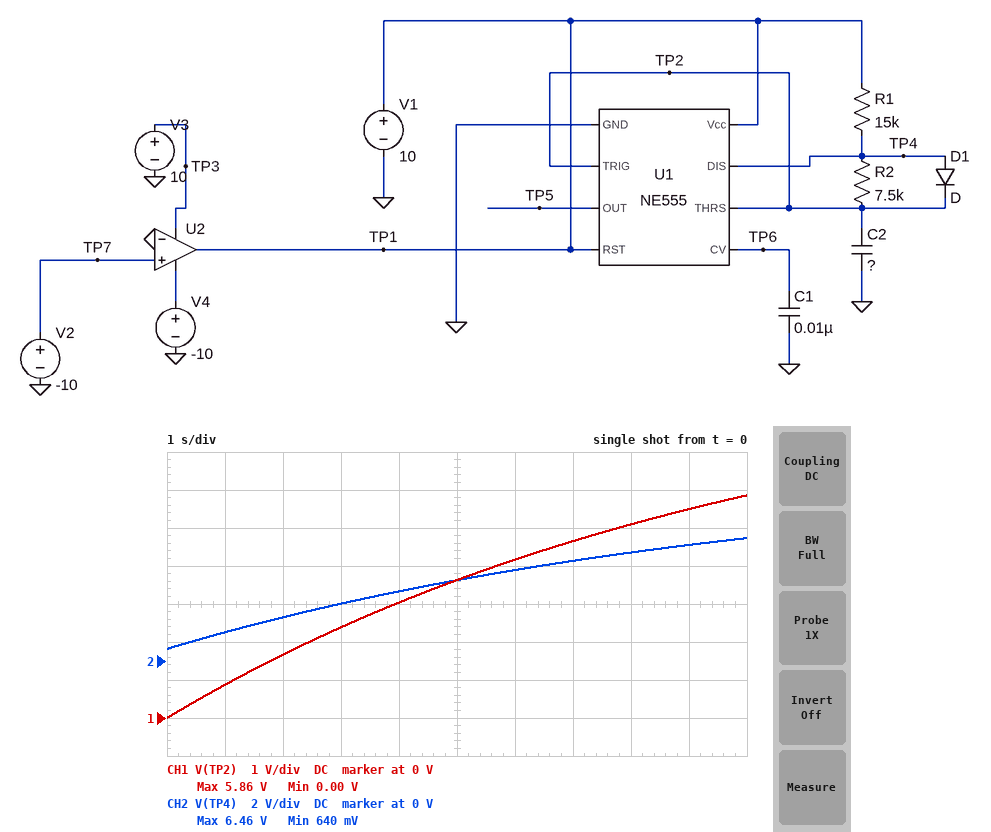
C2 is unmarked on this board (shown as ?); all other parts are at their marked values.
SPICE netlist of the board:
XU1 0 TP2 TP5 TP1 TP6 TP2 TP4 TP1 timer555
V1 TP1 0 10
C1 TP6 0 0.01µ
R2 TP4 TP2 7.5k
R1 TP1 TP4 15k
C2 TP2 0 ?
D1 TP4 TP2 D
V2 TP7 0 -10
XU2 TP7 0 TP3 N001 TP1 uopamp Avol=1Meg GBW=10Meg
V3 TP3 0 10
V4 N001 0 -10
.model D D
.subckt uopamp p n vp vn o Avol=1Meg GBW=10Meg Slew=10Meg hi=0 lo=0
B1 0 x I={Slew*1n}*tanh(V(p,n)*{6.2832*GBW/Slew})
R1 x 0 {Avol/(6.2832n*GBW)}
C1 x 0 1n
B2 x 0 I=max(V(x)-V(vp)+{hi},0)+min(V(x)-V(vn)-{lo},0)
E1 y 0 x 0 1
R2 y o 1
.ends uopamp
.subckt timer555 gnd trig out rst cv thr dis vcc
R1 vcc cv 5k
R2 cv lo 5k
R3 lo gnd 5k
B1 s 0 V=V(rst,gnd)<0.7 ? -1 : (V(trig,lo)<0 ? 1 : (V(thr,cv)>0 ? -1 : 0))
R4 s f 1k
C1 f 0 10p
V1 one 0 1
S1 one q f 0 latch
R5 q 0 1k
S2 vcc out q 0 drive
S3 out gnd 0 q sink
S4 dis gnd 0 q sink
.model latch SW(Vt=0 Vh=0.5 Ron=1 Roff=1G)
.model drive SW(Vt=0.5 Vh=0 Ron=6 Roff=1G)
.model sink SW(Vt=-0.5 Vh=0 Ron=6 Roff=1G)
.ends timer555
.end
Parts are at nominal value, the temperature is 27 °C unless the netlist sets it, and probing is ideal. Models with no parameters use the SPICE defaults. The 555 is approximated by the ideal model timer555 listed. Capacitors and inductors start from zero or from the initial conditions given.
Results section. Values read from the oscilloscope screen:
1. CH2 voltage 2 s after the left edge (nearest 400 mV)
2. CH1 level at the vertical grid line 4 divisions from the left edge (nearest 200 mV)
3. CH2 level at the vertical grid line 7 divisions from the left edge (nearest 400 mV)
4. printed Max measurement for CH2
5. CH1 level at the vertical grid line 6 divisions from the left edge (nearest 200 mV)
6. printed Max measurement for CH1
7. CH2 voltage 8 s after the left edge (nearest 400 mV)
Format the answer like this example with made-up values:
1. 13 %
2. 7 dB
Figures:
1. 2.4 V
2. 3.0 V
3. 5.2 V
4. 6.46 V
5. 4.2 V
6. 5.86 V
7. 5.6 V
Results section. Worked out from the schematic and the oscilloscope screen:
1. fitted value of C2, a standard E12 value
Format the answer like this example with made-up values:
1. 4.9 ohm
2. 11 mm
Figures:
1. 680 µF
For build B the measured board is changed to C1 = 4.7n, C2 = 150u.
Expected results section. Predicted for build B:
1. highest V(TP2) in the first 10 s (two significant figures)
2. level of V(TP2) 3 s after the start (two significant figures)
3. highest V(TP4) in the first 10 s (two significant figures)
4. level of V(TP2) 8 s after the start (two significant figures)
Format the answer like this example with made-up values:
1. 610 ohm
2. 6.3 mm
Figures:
1. 6.7 V
2. 5.5 V
3. 7.3 V
4. 6.4 V
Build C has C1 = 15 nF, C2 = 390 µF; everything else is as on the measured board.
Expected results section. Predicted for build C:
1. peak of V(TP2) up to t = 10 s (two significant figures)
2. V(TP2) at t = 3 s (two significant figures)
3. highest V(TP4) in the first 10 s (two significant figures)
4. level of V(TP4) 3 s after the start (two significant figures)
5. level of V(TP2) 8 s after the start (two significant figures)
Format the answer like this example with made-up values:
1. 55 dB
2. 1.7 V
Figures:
1. 6.7 V
2. 3.8 V
3. 7.3 V
4. 4.4 V
5. 5.2 V
